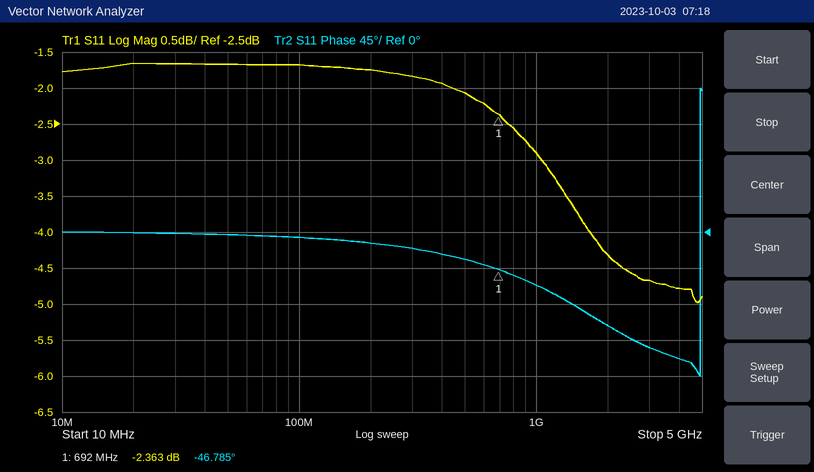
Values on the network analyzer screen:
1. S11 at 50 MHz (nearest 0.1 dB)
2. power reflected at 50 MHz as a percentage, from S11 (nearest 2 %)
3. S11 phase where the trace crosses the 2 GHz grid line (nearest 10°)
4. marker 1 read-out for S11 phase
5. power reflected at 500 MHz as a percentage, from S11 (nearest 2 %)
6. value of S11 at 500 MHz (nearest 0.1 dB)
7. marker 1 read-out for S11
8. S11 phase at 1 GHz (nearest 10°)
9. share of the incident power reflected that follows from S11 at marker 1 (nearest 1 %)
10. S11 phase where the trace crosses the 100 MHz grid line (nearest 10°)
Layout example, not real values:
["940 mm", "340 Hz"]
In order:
["-1.7 dB", "68 %", "-120°", "-46.785°", "62 %", "-2.1 dB", "-2.363 dB", "-70°", "58 %", "-10°"]
